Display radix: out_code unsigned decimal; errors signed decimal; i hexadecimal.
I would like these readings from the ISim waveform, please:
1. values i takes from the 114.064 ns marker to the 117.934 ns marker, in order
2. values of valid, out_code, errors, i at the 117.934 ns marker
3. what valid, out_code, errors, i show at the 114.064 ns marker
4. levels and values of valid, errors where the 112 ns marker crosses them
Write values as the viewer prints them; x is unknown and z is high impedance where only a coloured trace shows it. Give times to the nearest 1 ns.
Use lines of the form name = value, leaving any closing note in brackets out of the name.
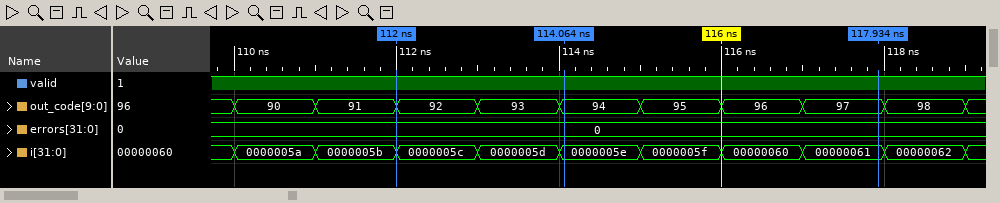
values i takes from the 114.064 ns marker to the 117.934 ns marker, in order = 0000005e, 0000005f, 00000060, 00000061
values of valid, out_code, errors, i at the 117.934 ns marker = valid=1, out_code=97, errors=0, i=00000061
what valid, out_code, errors, i show at the 114.064 ns marker = valid=1, out_code=94, errors=0, i=0000005e
levels and values of valid, errors where the 112 ns marker crosses them = valid=1, errors=0
